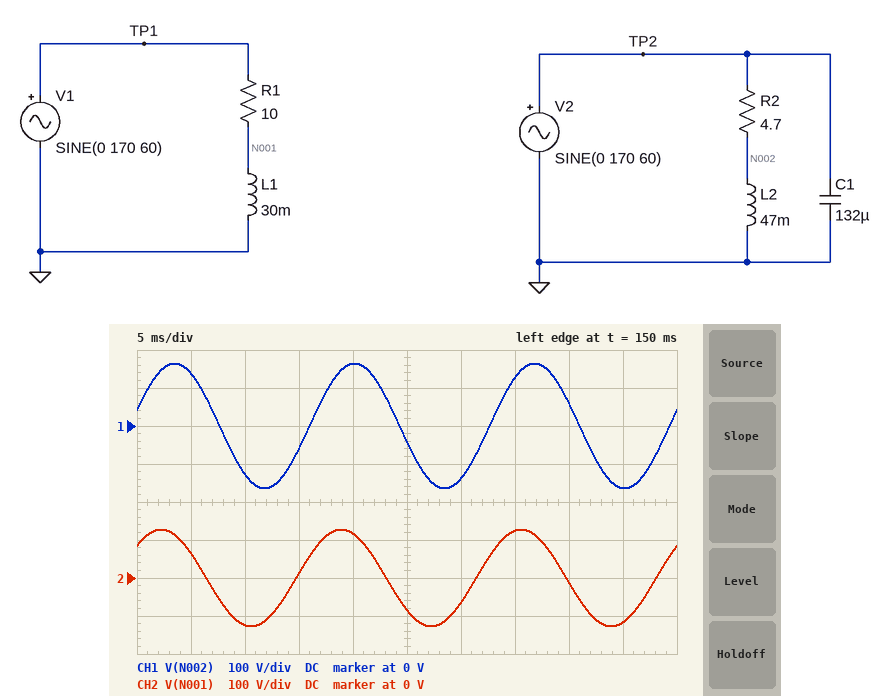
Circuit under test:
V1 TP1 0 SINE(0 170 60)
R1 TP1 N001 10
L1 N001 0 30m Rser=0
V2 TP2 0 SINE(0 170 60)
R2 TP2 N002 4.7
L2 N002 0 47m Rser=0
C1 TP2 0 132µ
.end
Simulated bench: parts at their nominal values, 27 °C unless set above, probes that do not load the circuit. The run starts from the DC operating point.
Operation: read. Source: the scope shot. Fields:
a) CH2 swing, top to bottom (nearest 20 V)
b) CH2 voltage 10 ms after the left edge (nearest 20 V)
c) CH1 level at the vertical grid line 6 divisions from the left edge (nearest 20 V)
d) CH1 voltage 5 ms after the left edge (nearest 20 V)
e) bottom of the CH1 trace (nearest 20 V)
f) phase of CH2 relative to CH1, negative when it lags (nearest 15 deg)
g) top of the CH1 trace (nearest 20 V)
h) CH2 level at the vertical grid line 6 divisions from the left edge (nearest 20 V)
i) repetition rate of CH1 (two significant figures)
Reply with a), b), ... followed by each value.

a) 260 V
b) -120 V
c) -140 V
d) 140 V
e) -160 V
f) 30 deg
g) 160 V
h) -60 V
i) 60 Hz
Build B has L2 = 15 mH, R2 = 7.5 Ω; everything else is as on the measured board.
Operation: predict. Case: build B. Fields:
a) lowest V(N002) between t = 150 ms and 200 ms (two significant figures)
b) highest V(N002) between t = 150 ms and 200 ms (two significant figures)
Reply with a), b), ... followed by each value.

a) -100 V
b) 100 V
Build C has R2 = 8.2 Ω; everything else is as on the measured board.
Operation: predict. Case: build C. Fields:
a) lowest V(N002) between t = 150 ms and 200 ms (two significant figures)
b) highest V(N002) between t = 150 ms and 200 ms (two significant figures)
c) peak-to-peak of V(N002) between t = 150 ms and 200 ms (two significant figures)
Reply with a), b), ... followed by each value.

a) -150 V
b) 150 V
c) 310 V
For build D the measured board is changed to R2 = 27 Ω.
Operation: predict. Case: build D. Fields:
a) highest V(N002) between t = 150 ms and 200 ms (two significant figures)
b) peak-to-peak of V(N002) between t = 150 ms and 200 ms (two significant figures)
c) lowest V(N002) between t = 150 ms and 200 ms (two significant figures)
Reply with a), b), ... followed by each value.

a) 93 V
b) 190 V
c) -93 V
